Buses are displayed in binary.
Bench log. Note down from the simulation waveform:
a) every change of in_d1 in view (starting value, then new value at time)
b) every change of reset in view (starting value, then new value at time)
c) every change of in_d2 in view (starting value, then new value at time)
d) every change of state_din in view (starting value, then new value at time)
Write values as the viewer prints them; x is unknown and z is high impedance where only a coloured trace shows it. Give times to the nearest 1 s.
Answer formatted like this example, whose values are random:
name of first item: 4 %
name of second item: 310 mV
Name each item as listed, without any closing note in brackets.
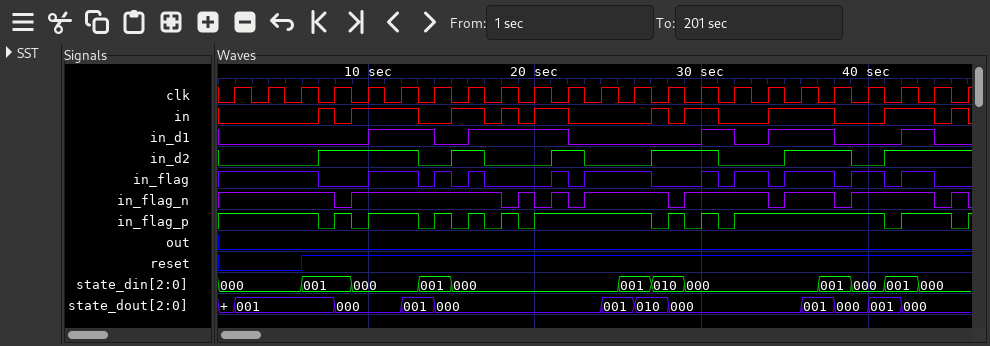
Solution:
every change of in_d1 in view: 0, 1 at 10 s, 0 at 14 s, 1 at 16 s, 0 at 22 s, 1 at 30 s, 0 at 32 s, 1 at 34 s, 0 at 38 s, 1 at 42 s, 0 at 44 s
every change of reset in view: 0, 1 at 6 s
every change of in_d2 in view: 0, 1 at 7 s, 0 at 13 s, 1 at 15 s, 0 at 17 s, 1 at 21 s, 0 at 23 s, 1 at 27 s, 0 at 31 s, 1 at 35 s, 0 at 39 s, 1 at 41 s
every change of state_din in view: 000, 001 at 6 s, 000 at 9 s, 001 at 13 s, 000 at 15 s, 001 at 25 s, 010 at 27 s, 000 at 29 s, 001 at 37 s, 000 at 39 s, 001 at 41 s, 000 at 43 s
